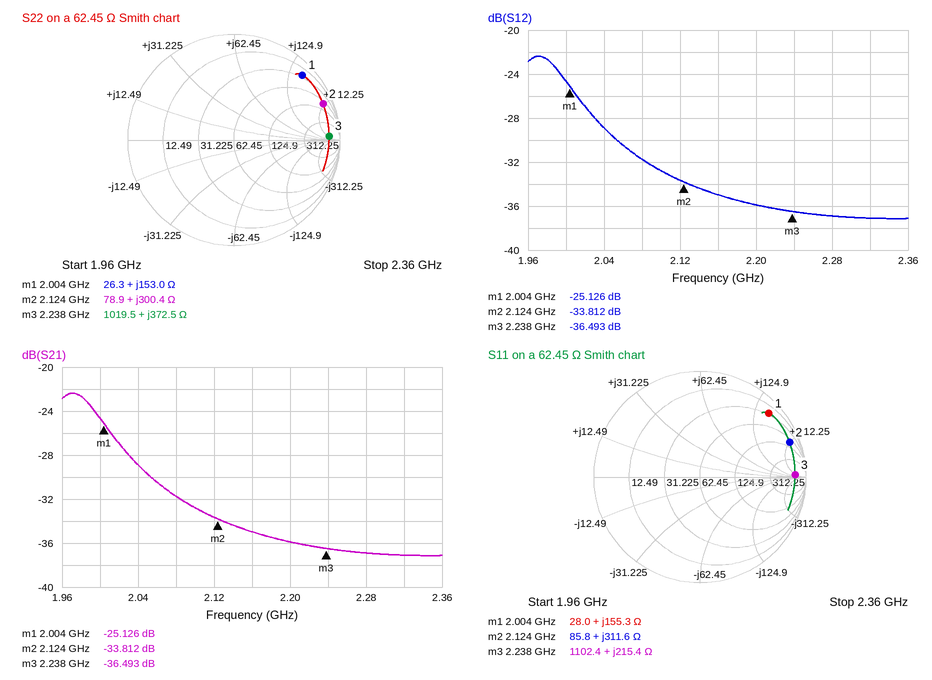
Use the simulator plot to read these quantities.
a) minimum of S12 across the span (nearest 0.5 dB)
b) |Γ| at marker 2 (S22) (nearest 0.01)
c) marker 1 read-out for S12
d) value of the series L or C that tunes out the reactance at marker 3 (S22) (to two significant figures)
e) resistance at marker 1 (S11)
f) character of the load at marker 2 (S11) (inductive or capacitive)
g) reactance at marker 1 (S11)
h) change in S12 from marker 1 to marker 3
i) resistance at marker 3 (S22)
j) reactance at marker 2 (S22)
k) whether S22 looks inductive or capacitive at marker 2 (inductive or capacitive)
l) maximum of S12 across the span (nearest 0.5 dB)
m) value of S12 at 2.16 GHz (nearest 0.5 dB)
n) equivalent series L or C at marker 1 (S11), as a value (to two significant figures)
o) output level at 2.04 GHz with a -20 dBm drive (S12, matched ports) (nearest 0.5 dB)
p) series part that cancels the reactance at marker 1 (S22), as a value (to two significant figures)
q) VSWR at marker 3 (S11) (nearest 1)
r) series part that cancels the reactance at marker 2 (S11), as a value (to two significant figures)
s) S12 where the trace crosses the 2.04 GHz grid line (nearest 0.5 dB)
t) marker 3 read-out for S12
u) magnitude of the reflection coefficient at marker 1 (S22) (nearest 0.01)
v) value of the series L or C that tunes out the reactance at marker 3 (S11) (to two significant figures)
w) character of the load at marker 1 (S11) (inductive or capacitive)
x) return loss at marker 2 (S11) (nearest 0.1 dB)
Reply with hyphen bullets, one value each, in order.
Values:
- -37.0 dB
- 0.91
- -25.126 dB
- 190 fF
- 28.0 Ω
- inductive
- +155.3 Ω
- -11.367 dB
- 1019.5 Ω
- +300.4 Ω
- inductive
- -22.5 dB
- -35.0 dB
- 12 nH
- -49.0 dBm
- 520 fF
- 18
- 240 fF
- -29.0 dB
- -36.493 dB
- 0.89
- 330 fF
- inductive
- 0.9 dB
